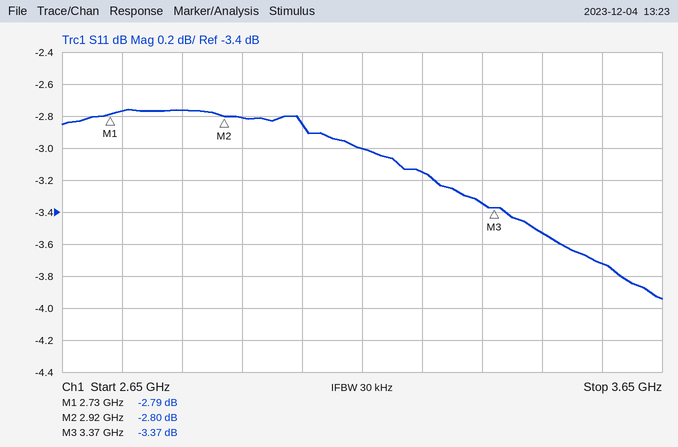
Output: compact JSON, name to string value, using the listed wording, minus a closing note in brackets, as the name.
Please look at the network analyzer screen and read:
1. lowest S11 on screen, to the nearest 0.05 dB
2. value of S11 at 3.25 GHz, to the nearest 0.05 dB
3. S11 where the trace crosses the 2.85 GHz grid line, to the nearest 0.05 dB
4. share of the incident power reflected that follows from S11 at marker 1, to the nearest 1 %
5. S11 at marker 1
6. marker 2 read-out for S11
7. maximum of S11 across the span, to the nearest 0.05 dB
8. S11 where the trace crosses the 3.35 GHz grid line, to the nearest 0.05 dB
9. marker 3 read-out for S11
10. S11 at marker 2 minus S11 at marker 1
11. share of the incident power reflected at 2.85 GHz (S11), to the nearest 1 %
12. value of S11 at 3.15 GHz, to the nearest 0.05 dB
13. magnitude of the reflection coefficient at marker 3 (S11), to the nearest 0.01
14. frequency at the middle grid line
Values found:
{"lowest S11 on screen, to the nearest 0.05 dB": "-3.95 dB", "value of S11 at 3.25 GHz, to the nearest 0.05 dB": "-3.15 dB", "S11 where the trace crosses the 2.85 GHz grid line, to the nearest 0.05 dB": "-2.75 dB", "share of the incident power reflected that follows from S11 at marker 1, to the nearest 1 %": "53 %", "S11 at marker 1": "-2.79 dB", "marker 2 read-out for S11": "-2.80 dB", "maximum of S11 across the span, to the nearest 0.05 dB": "-2.75 dB", "S11 where the trace crosses the 3.35 GHz grid line, to the nearest 0.05 dB": "-3.35 dB", "marker 3 read-out for S11": "-3.37 dB", "S11 at marker 2 minus S11 at marker 1": "-0.01 dB", "share of the incident power reflected at 2.85 GHz (S11), to the nearest 1 %": "53 %", "value of S11 at 3.15 GHz, to the nearest 0.05 dB": "-3.00 dB", "magnitude of the reflection coefficient at marker 3 (S11), to the nearest 0.01": "0.68", "frequency at the middle grid line": "3.15 GHz"}
